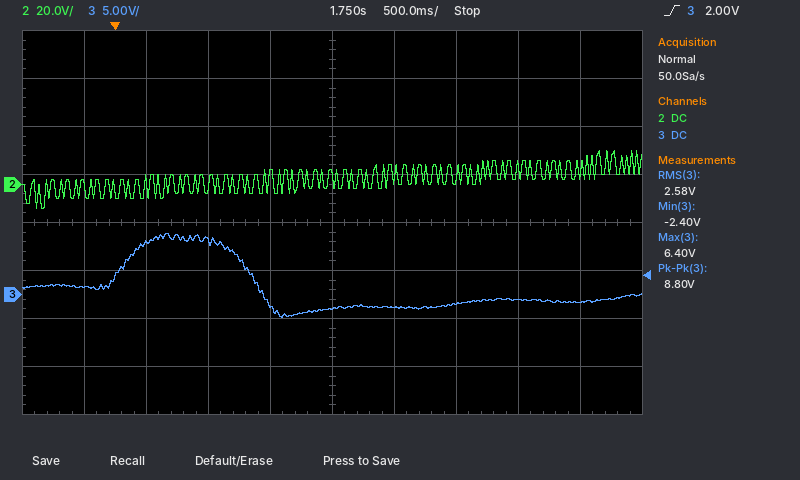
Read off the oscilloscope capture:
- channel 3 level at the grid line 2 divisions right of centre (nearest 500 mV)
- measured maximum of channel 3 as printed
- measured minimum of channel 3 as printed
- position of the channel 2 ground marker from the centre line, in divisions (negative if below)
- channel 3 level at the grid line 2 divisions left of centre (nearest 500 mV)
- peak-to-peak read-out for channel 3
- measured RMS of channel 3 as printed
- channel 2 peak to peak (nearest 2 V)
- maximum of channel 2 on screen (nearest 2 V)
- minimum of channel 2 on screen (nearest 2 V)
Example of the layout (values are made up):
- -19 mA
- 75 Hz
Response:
- -1.0 V
- 6.40 V
- -2.40 V
- +0.8 div
- 5.5 V
- 8.80 V
- 2.58 V
- 24 V
- 14 V
- -10 V
